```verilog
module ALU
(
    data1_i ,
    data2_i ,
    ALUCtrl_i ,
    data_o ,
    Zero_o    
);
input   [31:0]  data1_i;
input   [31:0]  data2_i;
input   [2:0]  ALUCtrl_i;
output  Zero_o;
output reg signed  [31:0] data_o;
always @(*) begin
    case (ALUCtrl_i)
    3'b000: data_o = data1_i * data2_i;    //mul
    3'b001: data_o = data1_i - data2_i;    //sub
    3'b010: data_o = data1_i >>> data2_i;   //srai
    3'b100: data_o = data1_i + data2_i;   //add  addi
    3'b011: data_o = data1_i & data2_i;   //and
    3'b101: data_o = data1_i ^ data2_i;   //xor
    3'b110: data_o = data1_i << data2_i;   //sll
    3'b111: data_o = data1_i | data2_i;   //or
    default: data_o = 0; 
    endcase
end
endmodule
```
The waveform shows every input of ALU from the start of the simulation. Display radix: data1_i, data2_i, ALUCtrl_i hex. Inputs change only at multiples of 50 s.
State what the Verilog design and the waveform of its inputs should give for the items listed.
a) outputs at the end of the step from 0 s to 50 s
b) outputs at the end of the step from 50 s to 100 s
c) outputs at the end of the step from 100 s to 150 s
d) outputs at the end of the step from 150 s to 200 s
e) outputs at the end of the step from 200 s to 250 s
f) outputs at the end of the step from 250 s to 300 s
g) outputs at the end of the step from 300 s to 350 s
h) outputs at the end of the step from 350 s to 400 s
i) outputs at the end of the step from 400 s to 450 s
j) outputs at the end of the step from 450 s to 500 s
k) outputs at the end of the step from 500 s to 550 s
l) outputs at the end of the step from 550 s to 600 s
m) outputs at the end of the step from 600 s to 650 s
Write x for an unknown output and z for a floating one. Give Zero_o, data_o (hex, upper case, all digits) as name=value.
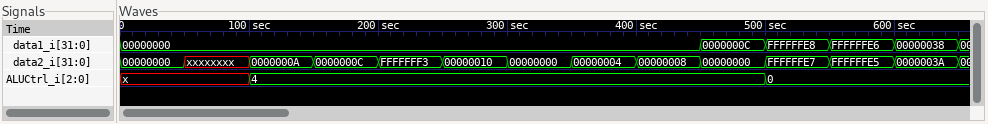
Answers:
Zero_o=z, data_o=00000000
Zero_o=z, data_o=00000000
Zero_o=z, data_o=0000000A
Zero_o=z, data_o=0000000C
Zero_o=z, data_o=FFFFFFF3
Zero_o=z, data_o=00000010
Zero_o=z, data_o=00000000
Zero_o=z, data_o=00000004
Zero_o=z, data_o=00000008
Zero_o=z, data_o=0000000C
Zero_o=z, data_o=00000258
Zero_o=z, data_o=000002BE
Zero_o=z, data_o=00000CB0
